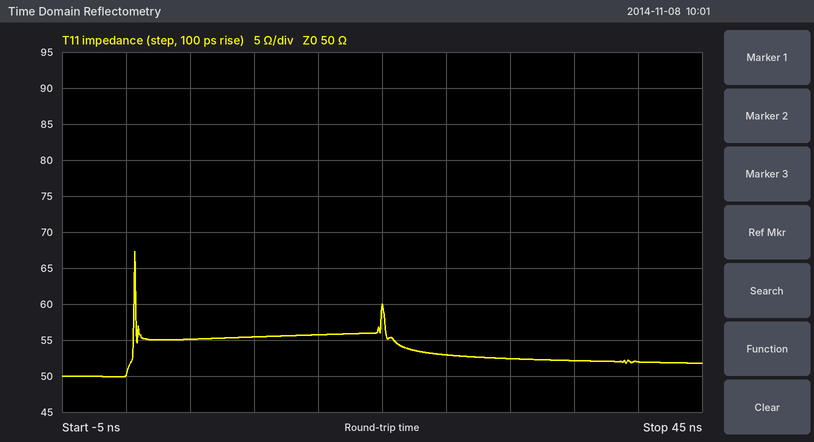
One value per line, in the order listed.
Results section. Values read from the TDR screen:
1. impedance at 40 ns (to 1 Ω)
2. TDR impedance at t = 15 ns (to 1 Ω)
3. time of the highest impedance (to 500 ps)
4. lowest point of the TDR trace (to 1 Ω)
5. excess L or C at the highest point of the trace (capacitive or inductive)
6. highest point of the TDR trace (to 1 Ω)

52 Ω
56 Ω
500 ps
50 Ω
inductive
67 Ω
